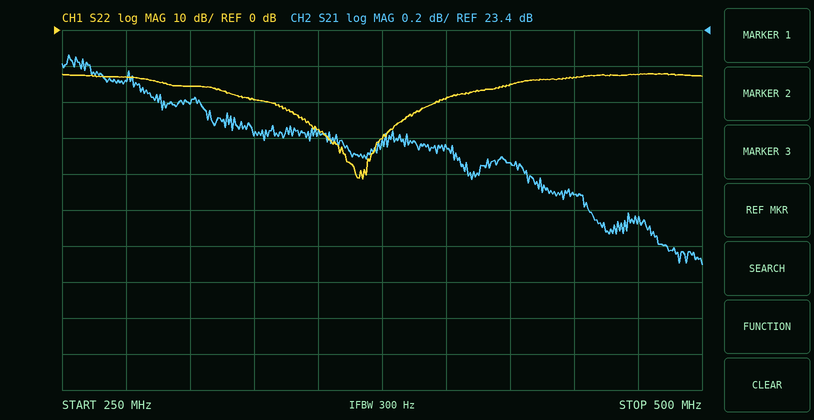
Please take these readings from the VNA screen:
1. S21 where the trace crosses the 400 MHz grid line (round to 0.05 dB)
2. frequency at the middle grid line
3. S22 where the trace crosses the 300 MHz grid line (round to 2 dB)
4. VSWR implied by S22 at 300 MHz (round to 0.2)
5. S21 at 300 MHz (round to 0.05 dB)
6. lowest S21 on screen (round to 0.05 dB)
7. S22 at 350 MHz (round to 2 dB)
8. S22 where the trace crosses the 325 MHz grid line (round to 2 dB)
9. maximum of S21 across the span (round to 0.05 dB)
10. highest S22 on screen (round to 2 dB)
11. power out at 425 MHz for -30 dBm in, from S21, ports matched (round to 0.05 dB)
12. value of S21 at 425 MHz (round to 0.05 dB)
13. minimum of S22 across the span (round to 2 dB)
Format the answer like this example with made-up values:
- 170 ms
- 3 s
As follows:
- 22.75 dB
- 375 MHz
- -16 dB
- 1.4
- 23.00 dB
- 22.10 dB
- -28 dB
- -20 dB
- 23.25 dB
- -12 dB
- -7.35 dBm
- 22.65 dB
- -42 dB
